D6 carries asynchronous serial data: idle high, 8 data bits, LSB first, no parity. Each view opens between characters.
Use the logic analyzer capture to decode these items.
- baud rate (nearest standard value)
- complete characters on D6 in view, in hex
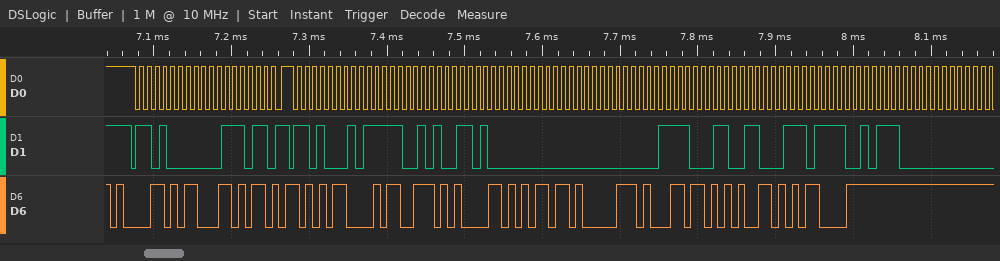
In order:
115200 baud
61, 63, 6B, 0D, 73, 61, 6D, 70, 6C, 65, 0D
